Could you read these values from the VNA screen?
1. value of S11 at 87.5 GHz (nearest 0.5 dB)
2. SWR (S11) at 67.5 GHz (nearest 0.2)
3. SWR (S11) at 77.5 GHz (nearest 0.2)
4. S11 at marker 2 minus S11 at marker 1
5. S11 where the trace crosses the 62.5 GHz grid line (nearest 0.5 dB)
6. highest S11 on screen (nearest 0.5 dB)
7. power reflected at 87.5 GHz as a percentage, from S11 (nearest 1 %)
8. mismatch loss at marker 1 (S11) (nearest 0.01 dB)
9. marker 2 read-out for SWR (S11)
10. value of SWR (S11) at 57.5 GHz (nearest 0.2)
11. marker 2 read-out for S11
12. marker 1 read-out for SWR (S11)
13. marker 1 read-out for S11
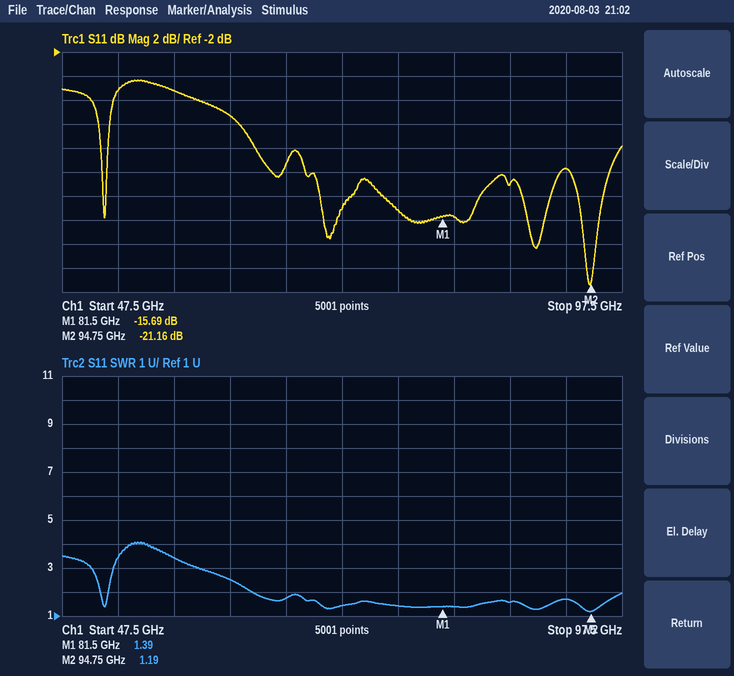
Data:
-13.0 dB
1.8
1.4
-5.47 dB
-7.5 dB
-4.5 dB
5 %
0.12 dB
1.19
3.4
-21.16 dB
1.39
-15.69 dB
